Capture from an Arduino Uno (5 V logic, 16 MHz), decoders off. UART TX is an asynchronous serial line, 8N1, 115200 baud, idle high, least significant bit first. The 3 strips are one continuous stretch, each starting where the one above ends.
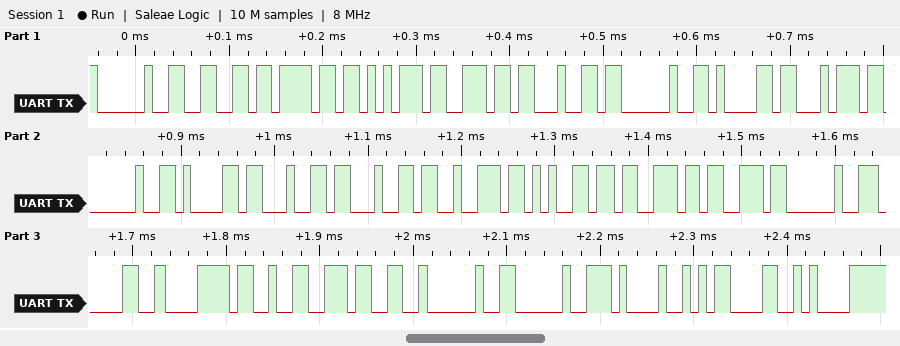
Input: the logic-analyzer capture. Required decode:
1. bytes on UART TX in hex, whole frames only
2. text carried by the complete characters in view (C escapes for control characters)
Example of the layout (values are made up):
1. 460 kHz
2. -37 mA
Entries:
1. 20 66 6F 75 6E 64 20 61 74 20 61 64 64 72 65 73 73 20 30 78 32 33 20 20 21 0D 0A
2. " found at address 0x23  !\r\n"
